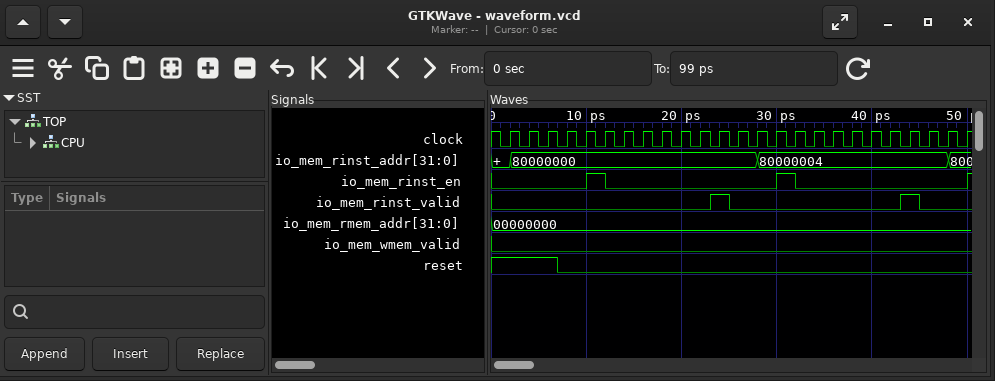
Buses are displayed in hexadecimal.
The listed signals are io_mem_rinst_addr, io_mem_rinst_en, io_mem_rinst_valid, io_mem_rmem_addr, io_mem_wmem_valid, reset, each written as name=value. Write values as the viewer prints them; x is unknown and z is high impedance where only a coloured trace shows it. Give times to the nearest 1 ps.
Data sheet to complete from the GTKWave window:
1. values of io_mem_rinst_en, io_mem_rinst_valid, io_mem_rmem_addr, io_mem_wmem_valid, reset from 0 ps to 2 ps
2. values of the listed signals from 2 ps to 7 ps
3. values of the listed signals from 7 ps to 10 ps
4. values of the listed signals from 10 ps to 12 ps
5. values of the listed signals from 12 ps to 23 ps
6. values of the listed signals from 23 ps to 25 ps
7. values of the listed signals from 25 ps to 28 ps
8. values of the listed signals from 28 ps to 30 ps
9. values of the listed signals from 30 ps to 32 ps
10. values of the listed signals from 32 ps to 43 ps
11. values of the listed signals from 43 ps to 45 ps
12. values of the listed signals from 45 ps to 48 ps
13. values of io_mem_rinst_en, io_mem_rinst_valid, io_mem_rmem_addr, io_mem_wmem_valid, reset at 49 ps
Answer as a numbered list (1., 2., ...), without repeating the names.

1. io_mem_rinst_en=0, io_mem_rinst_valid=0, io_mem_rmem_addr=00000000, io_mem_wmem_valid=0, reset=1
2. io_mem_rinst_addr=80000000, io_mem_rinst_en=0, io_mem_rinst_valid=0, io_mem_rmem_addr=00000000, io_mem_wmem_valid=0, reset=1
3. io_mem_rinst_addr=80000000, io_mem_rinst_en=0, io_mem_rinst_valid=0, io_mem_rmem_addr=00000000, io_mem_wmem_valid=0, reset=0
4. io_mem_rinst_addr=80000000, io_mem_rinst_en=1, io_mem_rinst_valid=0, io_mem_rmem_addr=00000000, io_mem_wmem_valid=0, reset=0
5. io_mem_rinst_addr=80000000, io_mem_rinst_en=0, io_mem_rinst_valid=0, io_mem_rmem_addr=00000000, io_mem_wmem_valid=0, reset=0
6. io_mem_rinst_addr=80000000, io_mem_rinst_en=0, io_mem_rinst_valid=1, io_mem_rmem_addr=00000000, io_mem_wmem_valid=0, reset=0
7. io_mem_rinst_addr=80000000, io_mem_rinst_en=0, io_mem_rinst_valid=0, io_mem_rmem_addr=00000000, io_mem_wmem_valid=0, reset=0
8. io_mem_rinst_addr=80000004, io_mem_rinst_en=0, io_mem_rinst_valid=0, io_mem_rmem_addr=00000000, io_mem_wmem_valid=0, reset=0
9. io_mem_rinst_addr=80000004, io_mem_rinst_en=1, io_mem_rinst_valid=0, io_mem_rmem_addr=00000000, io_mem_wmem_valid=0, reset=0
10. io_mem_rinst_addr=80000004, io_mem_rinst_en=0, io_mem_rinst_valid=0, io_mem_rmem_addr=00000000, io_mem_wmem_valid=0, reset=0
11. io_mem_rinst_addr=80000004, io_mem_rinst_en=0, io_mem_rinst_valid=1, io_mem_rmem_addr=00000000, io_mem_wmem_valid=0, reset=0
12. io_mem_rinst_addr=80000004, io_mem_rinst_en=0, io_mem_rinst_valid=0, io_mem_rmem_addr=00000000, io_mem_wmem_valid=0, reset=0
13. io_mem_rinst_en=0, io_mem_rinst_valid=0, io_mem_rmem_addr=00000000, io_mem_wmem_valid=0, reset=0
